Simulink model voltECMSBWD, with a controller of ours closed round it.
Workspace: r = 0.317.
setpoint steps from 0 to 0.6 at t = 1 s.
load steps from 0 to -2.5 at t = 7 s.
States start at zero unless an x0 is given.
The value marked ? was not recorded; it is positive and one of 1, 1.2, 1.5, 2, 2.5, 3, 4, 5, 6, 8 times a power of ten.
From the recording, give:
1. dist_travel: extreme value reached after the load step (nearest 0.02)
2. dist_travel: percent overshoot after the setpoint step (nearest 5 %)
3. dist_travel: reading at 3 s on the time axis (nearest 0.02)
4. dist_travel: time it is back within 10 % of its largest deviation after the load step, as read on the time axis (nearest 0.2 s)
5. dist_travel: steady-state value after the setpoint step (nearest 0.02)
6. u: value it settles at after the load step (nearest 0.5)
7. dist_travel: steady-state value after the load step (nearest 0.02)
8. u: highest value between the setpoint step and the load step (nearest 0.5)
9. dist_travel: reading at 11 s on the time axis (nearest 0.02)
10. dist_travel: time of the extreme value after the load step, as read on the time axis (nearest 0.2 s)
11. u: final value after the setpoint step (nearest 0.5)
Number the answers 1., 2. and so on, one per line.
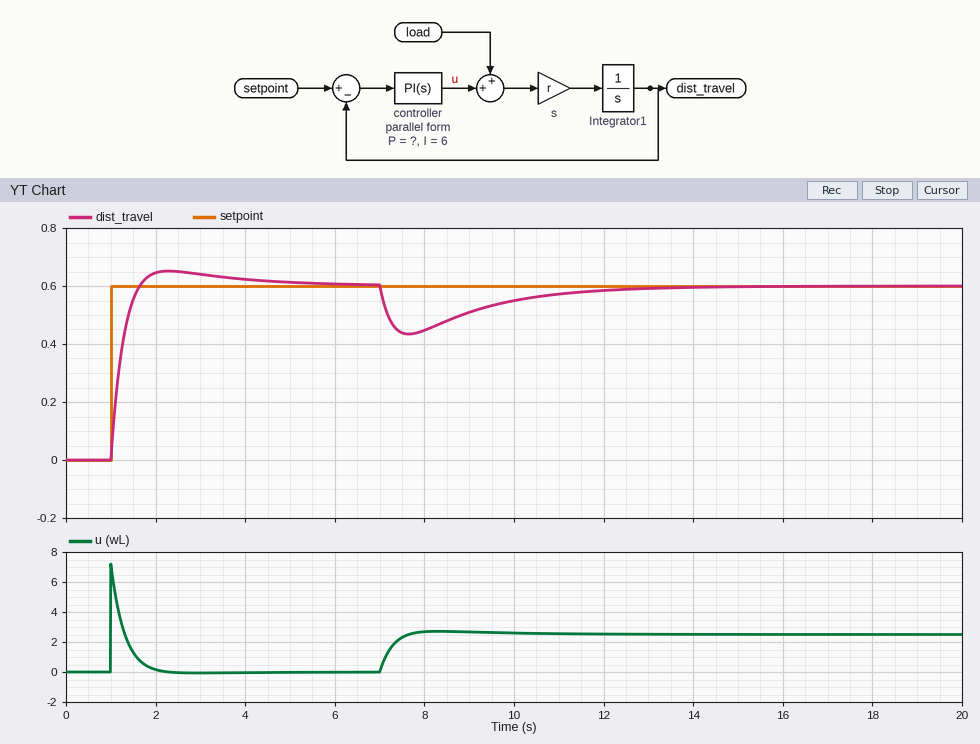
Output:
1. 0.44
2. 10 %
3. 0.64
4. 11.8 s
5. 0.60
6. 2.5
7. 0.60
8. 7.0
9. 0.58
10. 7.6 s
11. 0.0
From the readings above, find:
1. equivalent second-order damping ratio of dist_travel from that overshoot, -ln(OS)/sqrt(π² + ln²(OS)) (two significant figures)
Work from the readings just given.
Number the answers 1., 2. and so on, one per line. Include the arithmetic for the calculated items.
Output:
1. ln(0.1) = -2.303; 2.303 / sqrt(9.870 + 5.302) = 0.59
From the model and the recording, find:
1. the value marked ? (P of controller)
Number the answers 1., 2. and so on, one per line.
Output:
1. 12
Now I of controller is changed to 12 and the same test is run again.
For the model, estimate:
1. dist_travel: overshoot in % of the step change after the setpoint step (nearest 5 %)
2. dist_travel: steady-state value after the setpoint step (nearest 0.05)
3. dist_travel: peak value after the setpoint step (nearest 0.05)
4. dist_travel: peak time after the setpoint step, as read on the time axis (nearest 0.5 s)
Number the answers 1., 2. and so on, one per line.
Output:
1. 15 %
2. 0.60
3. 0.70
4. 2.0 s
